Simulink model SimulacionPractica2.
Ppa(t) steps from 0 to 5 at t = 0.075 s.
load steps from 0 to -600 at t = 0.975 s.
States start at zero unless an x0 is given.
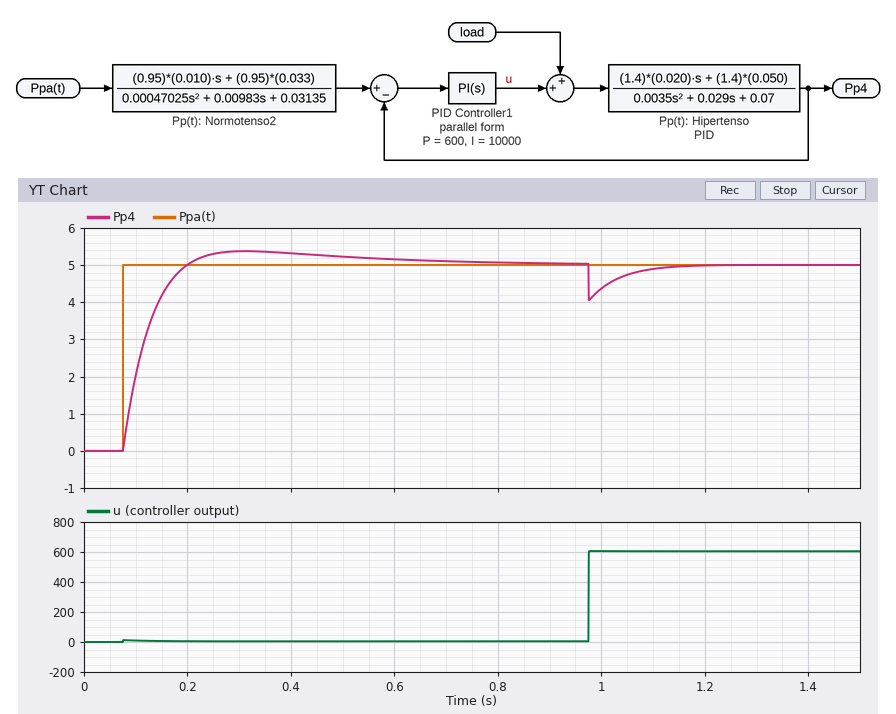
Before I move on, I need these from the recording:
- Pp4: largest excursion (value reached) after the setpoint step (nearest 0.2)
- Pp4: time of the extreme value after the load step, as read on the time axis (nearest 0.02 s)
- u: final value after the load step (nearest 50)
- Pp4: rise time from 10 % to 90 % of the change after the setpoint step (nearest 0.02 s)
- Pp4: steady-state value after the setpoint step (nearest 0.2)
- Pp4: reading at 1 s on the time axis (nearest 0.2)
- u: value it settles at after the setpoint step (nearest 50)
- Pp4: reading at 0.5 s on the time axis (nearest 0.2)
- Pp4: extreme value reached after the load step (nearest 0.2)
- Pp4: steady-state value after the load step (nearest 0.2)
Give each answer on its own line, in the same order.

5.4
0.98 s
600
0.08 s
5.0
4.4
0
5.2
4.0
5.0
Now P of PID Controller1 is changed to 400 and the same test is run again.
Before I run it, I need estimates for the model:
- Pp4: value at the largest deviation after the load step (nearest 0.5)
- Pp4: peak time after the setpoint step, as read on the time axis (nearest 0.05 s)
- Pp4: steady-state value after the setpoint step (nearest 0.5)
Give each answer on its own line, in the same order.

3.5
0.30 s
5.0
